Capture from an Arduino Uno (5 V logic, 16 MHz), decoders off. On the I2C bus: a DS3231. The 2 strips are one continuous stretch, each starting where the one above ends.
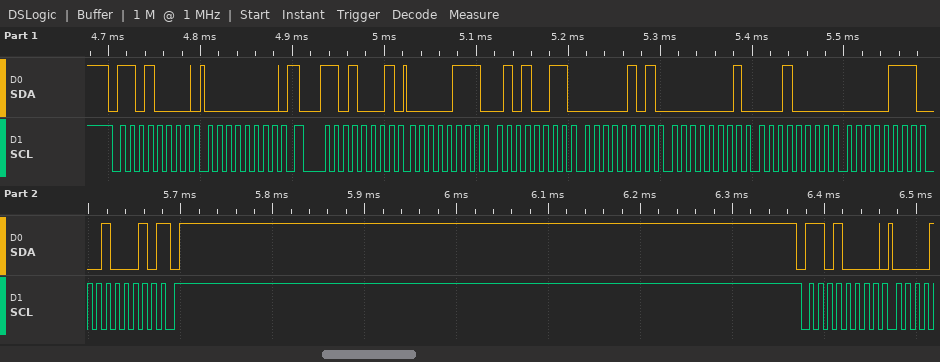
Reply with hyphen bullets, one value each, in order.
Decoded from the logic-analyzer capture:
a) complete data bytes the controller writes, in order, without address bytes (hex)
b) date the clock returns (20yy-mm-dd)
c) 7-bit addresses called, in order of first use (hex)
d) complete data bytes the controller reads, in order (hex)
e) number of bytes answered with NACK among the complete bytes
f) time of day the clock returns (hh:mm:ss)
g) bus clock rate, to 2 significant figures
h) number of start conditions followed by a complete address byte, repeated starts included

- 00
- 2022-07-10
- 0x68
- 07 53 05 01 10 07 22
- 1
- 05:53:07
- 100 kHz
- 3
